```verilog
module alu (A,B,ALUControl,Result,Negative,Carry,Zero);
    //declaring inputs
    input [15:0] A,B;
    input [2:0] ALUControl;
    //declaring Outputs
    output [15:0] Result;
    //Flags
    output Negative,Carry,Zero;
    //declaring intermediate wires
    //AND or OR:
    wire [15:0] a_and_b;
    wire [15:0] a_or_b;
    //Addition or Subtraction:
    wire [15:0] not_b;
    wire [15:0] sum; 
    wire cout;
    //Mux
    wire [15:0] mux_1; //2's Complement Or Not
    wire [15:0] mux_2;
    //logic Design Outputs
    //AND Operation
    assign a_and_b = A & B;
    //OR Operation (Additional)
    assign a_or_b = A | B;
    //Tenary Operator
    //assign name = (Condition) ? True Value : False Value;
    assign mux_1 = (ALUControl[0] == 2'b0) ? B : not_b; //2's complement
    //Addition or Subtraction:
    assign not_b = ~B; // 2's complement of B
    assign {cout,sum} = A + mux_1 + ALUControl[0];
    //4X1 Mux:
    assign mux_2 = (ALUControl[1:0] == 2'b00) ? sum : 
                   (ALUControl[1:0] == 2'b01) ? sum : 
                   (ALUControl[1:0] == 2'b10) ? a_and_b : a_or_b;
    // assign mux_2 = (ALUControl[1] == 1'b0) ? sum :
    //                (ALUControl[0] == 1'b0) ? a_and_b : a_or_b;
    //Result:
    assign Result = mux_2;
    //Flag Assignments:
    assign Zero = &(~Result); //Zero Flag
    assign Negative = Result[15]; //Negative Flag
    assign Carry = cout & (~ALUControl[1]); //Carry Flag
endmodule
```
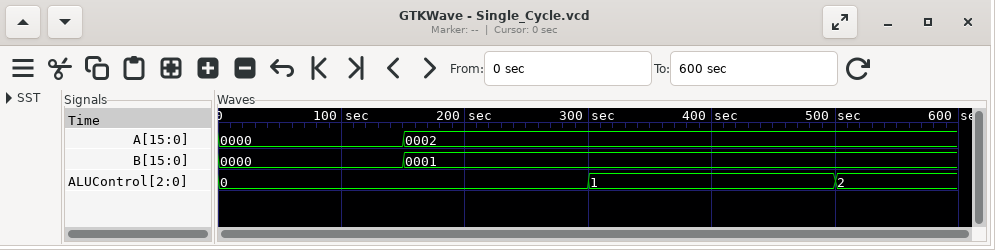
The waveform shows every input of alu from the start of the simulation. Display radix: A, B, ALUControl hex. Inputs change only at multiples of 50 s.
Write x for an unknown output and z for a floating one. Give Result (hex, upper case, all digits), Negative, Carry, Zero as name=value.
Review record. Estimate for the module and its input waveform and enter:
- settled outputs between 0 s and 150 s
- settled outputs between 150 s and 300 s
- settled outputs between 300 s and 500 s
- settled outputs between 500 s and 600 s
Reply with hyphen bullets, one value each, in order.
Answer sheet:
- Result=0000, Negative=0, Carry=0, Zero=1
- Result=0003, Negative=0, Carry=0, Zero=0
- Result=0001, Negative=0, Carry=1, Zero=0
- Result=0000, Negative=0, Carry=0, Zero=1
